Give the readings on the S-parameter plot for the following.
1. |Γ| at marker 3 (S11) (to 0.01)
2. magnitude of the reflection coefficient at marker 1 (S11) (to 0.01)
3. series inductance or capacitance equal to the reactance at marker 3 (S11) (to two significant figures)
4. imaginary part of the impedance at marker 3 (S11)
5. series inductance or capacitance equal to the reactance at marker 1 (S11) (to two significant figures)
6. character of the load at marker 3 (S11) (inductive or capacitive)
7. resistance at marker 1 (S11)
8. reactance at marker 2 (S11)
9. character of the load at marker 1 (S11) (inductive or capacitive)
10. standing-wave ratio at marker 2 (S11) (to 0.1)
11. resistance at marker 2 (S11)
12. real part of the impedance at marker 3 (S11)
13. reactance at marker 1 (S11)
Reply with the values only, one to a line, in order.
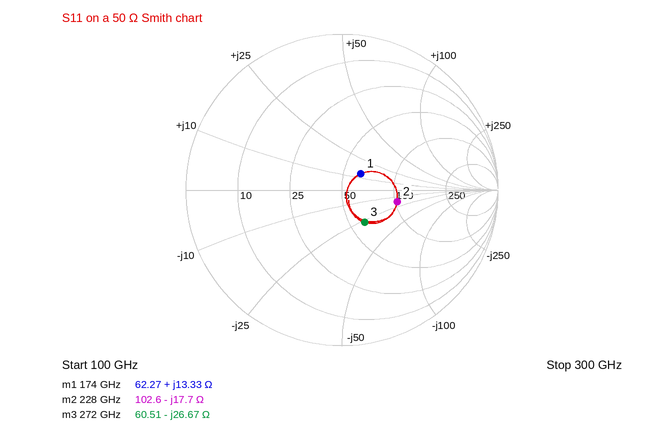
0.25
0.16
22 fF
-26.67 Ω
12 pH
capacitive
62.27 Ω
-17.7 Ω
inductive
2.1
102.6 Ω
60.51 Ω
+13.33 Ω
